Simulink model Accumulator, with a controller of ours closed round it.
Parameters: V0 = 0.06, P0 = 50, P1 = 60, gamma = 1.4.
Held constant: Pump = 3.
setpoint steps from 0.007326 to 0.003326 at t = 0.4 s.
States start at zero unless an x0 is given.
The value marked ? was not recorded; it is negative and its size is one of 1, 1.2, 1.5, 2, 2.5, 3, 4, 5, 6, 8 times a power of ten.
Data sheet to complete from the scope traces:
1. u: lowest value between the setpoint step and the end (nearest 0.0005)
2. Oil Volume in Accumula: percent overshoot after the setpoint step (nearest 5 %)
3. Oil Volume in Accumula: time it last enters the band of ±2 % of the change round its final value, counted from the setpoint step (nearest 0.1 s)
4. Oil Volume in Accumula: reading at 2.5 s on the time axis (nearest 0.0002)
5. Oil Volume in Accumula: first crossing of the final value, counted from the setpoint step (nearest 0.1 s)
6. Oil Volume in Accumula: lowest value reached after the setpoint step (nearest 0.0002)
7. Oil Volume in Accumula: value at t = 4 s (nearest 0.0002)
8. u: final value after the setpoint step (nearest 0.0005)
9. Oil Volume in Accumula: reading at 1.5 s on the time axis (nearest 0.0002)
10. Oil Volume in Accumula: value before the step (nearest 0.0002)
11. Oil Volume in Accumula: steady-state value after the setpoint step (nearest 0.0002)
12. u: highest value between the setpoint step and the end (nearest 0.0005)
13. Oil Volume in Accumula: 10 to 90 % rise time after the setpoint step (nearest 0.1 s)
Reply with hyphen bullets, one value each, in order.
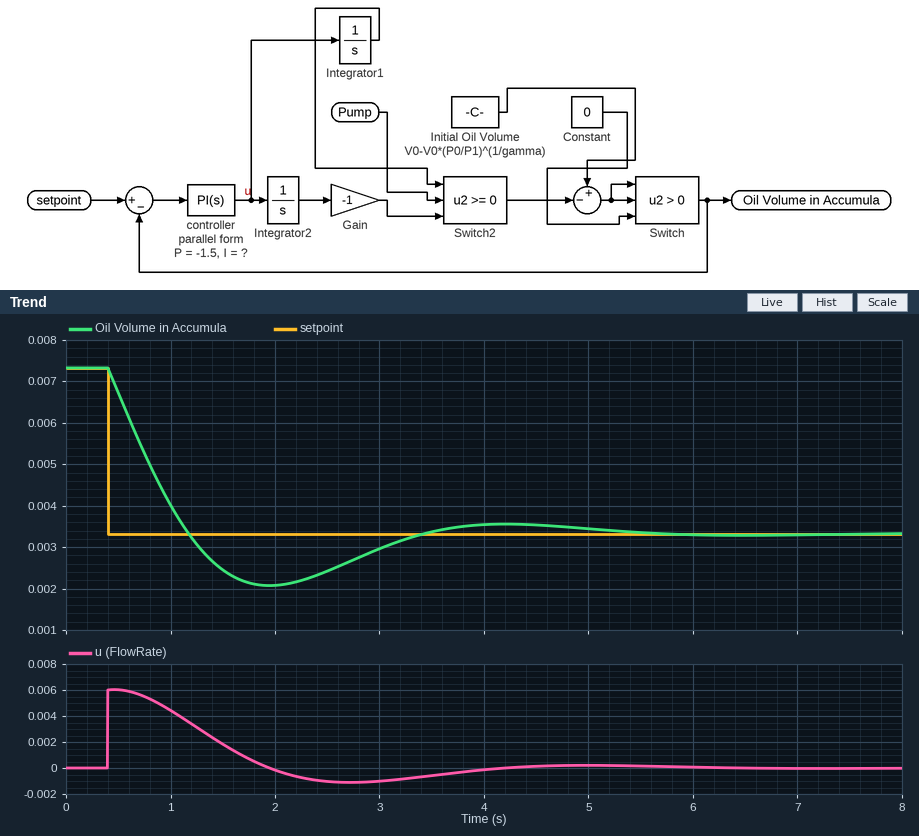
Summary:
- -0.0010
- 30 %
- 4.8 s
- 0.0024
- 0.8 s
- 0.0020
- 0.0036
- 0.0000
- 0.0024
- 0.0074
- 0.0034
- 0.0060
- 0.6 s
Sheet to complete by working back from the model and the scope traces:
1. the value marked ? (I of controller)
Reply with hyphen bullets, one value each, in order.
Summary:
- -2.5
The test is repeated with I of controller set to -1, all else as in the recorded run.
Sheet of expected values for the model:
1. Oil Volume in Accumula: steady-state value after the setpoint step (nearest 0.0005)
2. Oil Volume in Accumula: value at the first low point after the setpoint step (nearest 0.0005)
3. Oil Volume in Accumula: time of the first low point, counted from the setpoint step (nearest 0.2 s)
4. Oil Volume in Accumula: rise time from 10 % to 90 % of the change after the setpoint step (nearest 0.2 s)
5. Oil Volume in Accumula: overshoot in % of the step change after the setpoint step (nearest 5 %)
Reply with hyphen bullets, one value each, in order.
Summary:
- 0.0035
- 0.0025
- 2.2 s
- 0.8 s
- 20 %
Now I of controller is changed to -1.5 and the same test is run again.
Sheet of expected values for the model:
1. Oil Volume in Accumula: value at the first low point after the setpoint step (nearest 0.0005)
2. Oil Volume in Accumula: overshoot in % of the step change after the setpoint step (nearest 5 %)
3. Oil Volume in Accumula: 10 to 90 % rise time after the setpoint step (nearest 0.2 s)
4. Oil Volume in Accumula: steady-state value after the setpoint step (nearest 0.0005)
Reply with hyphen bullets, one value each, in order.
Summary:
- 0.0025
- 25 %
- 0.8 s
- 0.0035
